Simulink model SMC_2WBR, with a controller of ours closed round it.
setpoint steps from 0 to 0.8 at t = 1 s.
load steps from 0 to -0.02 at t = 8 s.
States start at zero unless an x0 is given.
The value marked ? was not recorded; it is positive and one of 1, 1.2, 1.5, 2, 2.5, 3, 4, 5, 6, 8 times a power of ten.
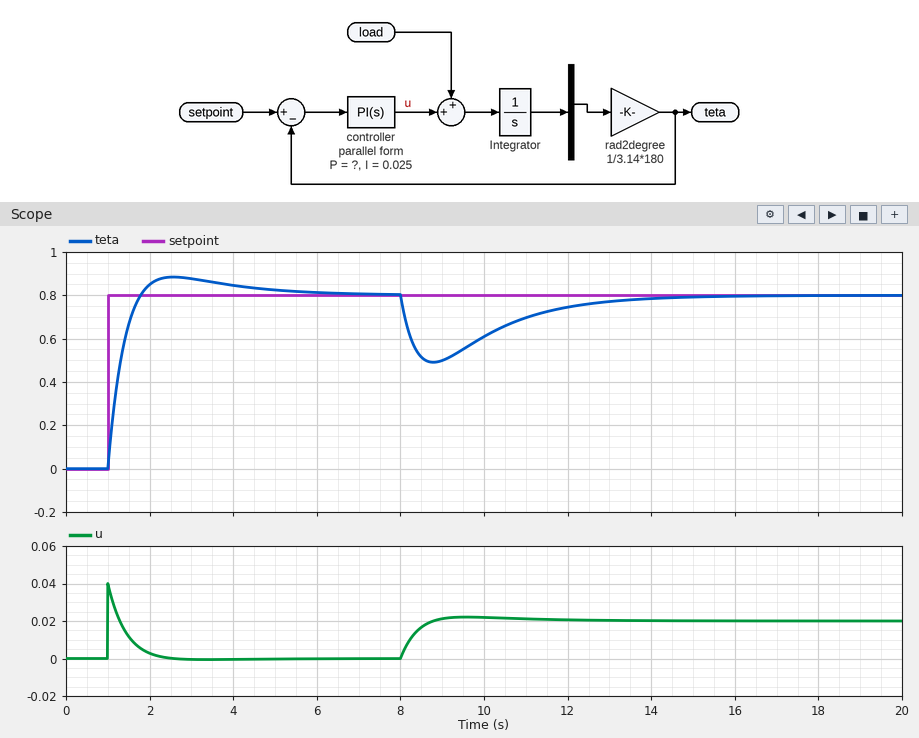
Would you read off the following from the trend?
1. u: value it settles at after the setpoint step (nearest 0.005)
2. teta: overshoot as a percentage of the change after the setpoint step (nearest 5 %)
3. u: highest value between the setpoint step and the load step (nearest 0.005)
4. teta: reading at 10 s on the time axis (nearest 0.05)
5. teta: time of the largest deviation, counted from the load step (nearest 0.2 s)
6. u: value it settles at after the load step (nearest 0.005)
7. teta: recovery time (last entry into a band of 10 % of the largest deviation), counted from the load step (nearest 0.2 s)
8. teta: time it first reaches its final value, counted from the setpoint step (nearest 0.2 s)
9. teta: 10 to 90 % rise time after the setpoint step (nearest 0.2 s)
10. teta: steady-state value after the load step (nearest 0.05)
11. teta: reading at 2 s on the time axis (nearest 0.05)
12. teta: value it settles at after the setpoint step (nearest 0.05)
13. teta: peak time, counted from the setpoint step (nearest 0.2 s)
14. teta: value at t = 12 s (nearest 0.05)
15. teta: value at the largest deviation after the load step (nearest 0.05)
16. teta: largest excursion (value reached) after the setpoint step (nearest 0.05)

0.000
10 %
0.040
0.60
0.8 s
0.020
4.8 s
0.8 s
0.6 s
0.80
0.85
0.80
1.6 s
0.75
0.50
0.90
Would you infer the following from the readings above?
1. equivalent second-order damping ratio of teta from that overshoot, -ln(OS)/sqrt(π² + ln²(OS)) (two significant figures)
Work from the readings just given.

0.59
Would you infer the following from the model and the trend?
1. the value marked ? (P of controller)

0.05
